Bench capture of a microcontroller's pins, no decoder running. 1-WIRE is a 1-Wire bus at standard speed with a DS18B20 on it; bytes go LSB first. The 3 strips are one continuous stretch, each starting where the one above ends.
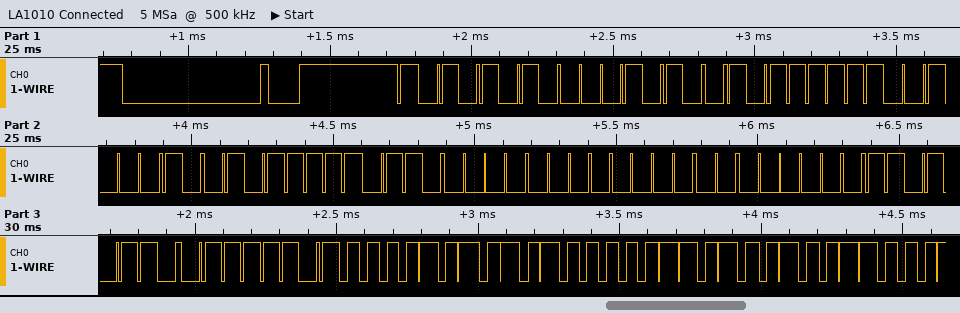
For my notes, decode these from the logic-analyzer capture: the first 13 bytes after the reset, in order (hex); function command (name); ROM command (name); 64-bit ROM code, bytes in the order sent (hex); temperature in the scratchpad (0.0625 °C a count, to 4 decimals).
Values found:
55 28 FD 44 FA 06 00 00 6B BE 50 05 4B
Read Scratchpad
Match ROM
28 FD 44 FA 06 00 00 6B
85.0000 °C
